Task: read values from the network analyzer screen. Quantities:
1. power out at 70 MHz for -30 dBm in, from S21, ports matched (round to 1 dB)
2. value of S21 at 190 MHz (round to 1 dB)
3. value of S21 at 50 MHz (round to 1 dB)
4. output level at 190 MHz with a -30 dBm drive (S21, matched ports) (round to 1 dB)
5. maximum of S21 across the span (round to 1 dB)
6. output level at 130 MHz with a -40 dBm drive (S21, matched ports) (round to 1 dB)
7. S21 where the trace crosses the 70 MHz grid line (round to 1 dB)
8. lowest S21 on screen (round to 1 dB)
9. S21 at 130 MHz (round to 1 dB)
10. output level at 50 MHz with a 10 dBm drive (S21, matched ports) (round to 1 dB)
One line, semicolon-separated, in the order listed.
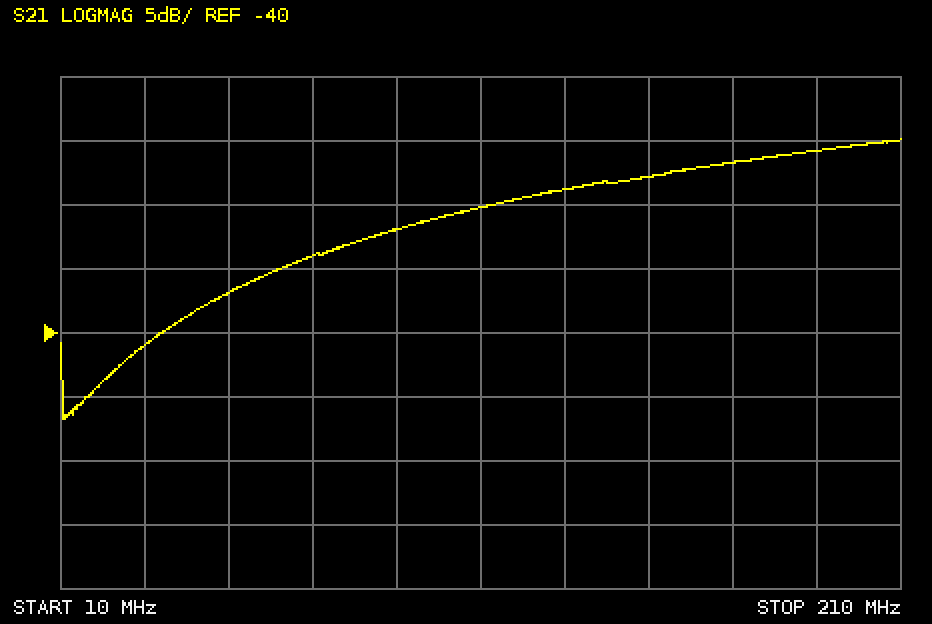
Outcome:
-64 dBm; -26 dB; -37 dB; -56 dBm; -25 dB; -69 dBm; -34 dB; -47 dB; -29 dB; -27 dBm
